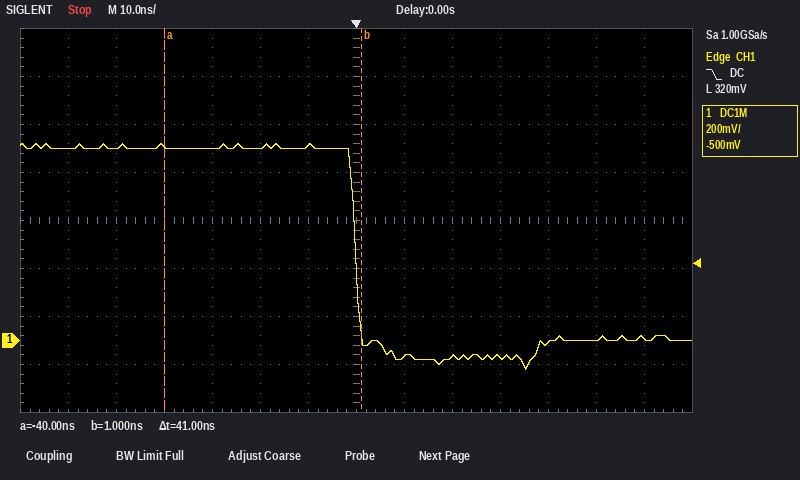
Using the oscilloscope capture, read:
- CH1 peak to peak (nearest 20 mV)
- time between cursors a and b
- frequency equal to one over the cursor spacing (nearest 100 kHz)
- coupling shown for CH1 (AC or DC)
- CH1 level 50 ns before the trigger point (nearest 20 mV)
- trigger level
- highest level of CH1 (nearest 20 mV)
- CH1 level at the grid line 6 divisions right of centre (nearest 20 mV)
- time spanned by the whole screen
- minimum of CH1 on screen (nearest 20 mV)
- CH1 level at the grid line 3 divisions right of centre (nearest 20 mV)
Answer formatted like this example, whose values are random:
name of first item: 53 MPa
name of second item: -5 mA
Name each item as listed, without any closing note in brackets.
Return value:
CH1 peak to peak: 940 mV
time between cursors a and b: 41 ns
frequency equal to one over the cursor spacing: 24.4 MHz
coupling shown for CH1: DC
CH1 level 50 ns before the trigger point: 800 mV
trigger level: 320 mV
highest level of CH1: 820 mV
CH1 level at the grid line 6 divisions right of centre: 0 mV
time spanned by the whole screen: 140 ns
minimum of CH1 on screen: -120 mV
CH1 level at the grid line 3 divisions right of centre: -80 mV
